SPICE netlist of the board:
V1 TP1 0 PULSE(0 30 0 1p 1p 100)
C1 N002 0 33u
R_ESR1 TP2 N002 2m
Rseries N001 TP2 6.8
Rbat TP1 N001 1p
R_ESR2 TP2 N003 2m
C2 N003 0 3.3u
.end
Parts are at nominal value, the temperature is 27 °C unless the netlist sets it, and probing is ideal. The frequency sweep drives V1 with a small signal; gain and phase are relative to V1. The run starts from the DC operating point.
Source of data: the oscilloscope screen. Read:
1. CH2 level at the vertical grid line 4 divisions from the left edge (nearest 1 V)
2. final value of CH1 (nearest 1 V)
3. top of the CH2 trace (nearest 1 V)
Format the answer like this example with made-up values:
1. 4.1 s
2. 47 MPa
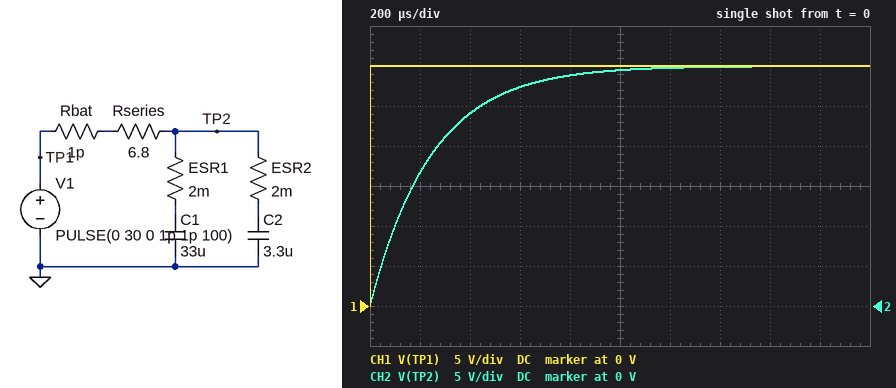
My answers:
1. 29 V
2. 30 V
3. 30 V
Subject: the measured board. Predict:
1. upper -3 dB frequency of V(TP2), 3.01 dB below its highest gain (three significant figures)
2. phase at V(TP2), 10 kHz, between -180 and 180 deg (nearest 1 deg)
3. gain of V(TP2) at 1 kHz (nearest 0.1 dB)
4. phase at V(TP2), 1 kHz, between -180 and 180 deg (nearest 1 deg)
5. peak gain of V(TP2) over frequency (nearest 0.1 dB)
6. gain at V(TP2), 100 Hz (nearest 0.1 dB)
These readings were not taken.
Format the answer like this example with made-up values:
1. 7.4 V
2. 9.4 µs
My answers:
1. 645 Hz
2. -86 deg
3. -5.3 dB
4. -57 deg
5. 0 dB
6. -0.1 dB
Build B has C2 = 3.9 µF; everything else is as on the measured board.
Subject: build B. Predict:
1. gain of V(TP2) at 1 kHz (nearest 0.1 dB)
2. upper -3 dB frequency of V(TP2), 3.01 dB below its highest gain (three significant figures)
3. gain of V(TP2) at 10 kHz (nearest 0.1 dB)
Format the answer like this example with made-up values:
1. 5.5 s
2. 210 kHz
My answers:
1. -5.4 dB
2. 634 Hz
3. -24.0 dB
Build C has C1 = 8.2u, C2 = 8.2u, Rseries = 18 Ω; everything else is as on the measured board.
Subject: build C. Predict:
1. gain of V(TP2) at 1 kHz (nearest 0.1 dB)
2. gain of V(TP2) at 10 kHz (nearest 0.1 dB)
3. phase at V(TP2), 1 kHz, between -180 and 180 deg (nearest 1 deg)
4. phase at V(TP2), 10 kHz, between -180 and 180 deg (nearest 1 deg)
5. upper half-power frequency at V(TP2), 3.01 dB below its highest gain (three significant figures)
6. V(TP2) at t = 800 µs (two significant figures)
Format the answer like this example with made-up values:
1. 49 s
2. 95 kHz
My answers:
1. -6.5 dB
2. -25.4 dB
3. -62 deg
4. -87 deg
5. 539 Hz
6. 28 V
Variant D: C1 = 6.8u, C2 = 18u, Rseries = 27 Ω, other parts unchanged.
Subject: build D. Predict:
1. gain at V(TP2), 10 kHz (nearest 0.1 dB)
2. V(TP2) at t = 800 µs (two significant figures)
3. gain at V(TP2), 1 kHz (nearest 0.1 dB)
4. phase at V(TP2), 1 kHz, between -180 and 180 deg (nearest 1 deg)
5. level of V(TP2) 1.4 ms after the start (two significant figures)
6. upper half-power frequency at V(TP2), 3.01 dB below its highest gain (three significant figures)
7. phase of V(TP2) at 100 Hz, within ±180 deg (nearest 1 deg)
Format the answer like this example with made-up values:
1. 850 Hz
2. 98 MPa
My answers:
1. -32.5 dB
2. 21 V
3. -12.7 dB
4. -77 deg
5. 26 V
6. 238 Hz
7. -23 deg
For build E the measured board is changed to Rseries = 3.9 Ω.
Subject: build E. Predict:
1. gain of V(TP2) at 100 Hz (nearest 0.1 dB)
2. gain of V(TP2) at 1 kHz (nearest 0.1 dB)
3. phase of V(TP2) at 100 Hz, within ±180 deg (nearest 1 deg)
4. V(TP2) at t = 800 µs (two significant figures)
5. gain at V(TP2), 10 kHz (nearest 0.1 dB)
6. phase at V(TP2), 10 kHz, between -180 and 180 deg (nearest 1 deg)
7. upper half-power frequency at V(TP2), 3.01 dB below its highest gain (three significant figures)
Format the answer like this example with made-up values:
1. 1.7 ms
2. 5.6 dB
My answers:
1. 0 dB
2. -2.5 dB
3. -5 deg
4. 30 V
5. -19.0 dB
6. -83 deg
7. 1.12 kHz
